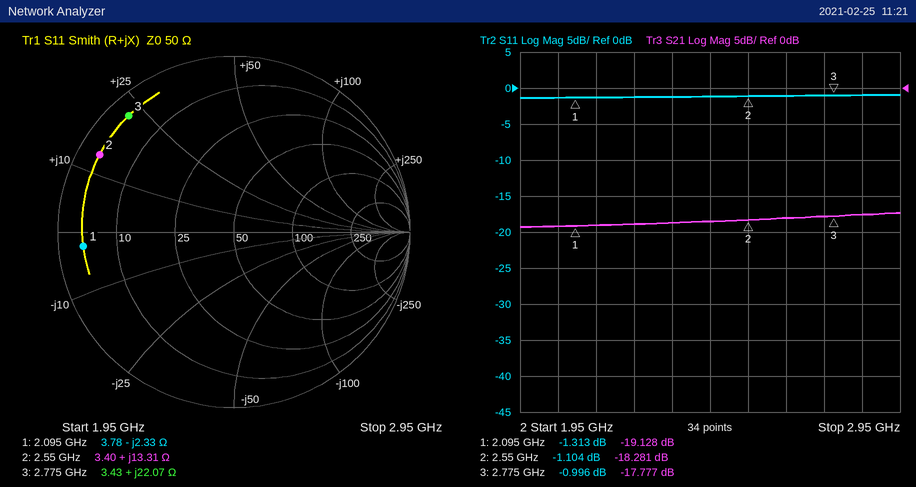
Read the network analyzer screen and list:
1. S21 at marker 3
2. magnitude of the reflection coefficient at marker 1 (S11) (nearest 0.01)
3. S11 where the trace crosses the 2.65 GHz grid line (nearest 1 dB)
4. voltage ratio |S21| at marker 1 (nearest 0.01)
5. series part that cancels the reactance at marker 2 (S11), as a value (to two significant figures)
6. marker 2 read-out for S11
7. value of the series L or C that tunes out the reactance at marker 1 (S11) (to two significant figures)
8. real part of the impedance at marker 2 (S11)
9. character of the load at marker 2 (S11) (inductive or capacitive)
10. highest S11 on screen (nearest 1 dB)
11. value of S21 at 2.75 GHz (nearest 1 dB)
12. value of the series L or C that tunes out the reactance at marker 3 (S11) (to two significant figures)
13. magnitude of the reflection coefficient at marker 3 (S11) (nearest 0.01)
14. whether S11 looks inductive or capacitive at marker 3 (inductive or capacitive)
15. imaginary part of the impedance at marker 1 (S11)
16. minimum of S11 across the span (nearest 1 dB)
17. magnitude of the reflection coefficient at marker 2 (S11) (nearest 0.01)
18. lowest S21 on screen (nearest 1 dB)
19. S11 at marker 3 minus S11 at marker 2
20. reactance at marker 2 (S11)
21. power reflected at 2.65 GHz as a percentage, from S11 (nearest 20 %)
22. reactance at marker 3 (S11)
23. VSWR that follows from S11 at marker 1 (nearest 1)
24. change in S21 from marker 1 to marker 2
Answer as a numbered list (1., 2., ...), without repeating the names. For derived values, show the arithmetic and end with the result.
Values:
1. -17.777 dB
2. 0.86
3. -1 dB
4. 10^(-19.128/20) ≈ 0.11
5. C = 1/(2π × 2.55 GHz × 13.31 Ω) ≈ 4.7 pF
6. -1.104 dB
7. L = 2.33 Ω/(2π × 2.095 GHz) ≈ 177 pH, so 180 pH to two significant figures
8. 3.40 Ω
9. inductive
10. -1 dB
11. -18 dB
12. C = 1/(2π × 2.775 GHz × 22.07 Ω) ≈ 2.6 pF
13. 10^(-0.996/20) ≈ 0.89
14. inductive
15. -2.33 Ω
16. -1 dB
17. 0.88
18. -19 dB
19. -0.996 − (-1.104) = 0.108 dB
20. +13.31 Ω
21. 10^(-1/10) ≈ 79.4 %, so 80 % to the nearest 20 %
22. +22.07 Ω
23. (1 + 0.8597)/(1 − 0.8597) ≈ 13
24. -18.281 − (-19.128) = 0.847 dB
